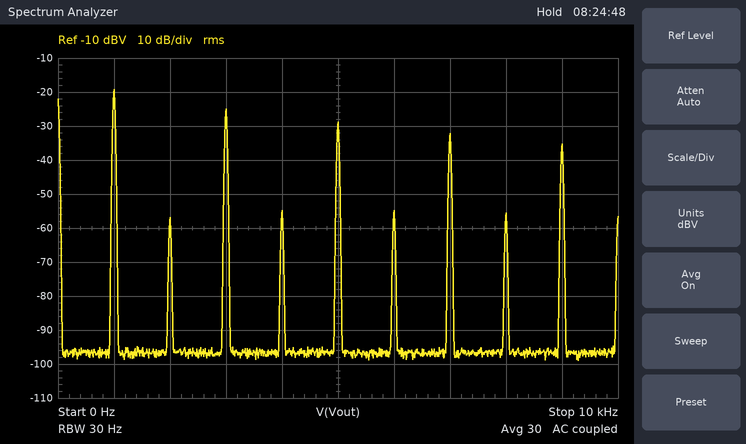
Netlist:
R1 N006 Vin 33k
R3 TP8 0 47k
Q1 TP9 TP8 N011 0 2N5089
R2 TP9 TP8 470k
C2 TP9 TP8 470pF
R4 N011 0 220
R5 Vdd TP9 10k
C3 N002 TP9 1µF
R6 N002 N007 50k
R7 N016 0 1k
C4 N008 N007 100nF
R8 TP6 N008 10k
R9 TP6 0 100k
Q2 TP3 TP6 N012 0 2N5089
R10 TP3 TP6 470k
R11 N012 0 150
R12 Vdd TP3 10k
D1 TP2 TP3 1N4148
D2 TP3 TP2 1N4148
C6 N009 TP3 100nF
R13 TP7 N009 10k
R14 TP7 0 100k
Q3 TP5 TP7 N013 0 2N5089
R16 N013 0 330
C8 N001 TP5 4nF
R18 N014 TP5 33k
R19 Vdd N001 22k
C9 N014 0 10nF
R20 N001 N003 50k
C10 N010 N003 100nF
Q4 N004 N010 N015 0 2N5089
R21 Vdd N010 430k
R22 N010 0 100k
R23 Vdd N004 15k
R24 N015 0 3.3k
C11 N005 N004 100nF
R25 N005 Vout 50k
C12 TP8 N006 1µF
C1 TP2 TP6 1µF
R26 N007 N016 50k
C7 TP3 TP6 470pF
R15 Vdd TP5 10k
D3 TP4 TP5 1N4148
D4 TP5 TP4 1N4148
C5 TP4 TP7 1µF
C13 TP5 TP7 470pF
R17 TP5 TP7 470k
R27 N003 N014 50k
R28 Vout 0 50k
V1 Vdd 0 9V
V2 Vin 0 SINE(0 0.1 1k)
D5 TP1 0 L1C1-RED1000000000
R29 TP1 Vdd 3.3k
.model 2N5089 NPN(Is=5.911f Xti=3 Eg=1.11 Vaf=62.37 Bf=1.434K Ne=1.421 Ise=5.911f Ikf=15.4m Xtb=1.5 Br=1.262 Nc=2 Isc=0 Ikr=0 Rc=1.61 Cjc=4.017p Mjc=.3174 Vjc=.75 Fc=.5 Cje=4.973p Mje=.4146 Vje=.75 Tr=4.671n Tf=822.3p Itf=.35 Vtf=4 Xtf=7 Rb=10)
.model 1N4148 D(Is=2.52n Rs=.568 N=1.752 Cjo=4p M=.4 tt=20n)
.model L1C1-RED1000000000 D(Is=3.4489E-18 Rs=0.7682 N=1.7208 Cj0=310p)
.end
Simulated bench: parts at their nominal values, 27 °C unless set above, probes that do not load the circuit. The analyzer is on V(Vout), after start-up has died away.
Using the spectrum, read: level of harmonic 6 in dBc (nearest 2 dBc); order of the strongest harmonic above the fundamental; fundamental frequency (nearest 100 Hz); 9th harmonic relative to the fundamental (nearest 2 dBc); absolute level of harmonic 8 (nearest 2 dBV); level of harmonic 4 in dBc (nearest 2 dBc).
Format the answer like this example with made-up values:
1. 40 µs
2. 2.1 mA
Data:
1. -36 dBc
2. 3
3. 1.0 kHz
4. -16 dBc
5. -56 dBV
6. -36 dBc
